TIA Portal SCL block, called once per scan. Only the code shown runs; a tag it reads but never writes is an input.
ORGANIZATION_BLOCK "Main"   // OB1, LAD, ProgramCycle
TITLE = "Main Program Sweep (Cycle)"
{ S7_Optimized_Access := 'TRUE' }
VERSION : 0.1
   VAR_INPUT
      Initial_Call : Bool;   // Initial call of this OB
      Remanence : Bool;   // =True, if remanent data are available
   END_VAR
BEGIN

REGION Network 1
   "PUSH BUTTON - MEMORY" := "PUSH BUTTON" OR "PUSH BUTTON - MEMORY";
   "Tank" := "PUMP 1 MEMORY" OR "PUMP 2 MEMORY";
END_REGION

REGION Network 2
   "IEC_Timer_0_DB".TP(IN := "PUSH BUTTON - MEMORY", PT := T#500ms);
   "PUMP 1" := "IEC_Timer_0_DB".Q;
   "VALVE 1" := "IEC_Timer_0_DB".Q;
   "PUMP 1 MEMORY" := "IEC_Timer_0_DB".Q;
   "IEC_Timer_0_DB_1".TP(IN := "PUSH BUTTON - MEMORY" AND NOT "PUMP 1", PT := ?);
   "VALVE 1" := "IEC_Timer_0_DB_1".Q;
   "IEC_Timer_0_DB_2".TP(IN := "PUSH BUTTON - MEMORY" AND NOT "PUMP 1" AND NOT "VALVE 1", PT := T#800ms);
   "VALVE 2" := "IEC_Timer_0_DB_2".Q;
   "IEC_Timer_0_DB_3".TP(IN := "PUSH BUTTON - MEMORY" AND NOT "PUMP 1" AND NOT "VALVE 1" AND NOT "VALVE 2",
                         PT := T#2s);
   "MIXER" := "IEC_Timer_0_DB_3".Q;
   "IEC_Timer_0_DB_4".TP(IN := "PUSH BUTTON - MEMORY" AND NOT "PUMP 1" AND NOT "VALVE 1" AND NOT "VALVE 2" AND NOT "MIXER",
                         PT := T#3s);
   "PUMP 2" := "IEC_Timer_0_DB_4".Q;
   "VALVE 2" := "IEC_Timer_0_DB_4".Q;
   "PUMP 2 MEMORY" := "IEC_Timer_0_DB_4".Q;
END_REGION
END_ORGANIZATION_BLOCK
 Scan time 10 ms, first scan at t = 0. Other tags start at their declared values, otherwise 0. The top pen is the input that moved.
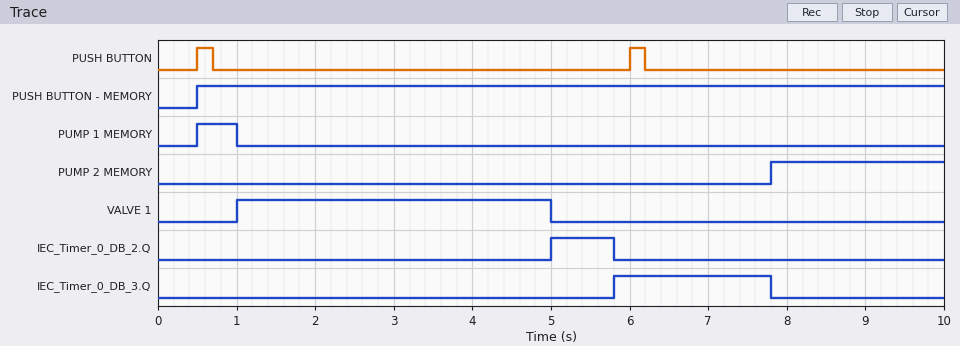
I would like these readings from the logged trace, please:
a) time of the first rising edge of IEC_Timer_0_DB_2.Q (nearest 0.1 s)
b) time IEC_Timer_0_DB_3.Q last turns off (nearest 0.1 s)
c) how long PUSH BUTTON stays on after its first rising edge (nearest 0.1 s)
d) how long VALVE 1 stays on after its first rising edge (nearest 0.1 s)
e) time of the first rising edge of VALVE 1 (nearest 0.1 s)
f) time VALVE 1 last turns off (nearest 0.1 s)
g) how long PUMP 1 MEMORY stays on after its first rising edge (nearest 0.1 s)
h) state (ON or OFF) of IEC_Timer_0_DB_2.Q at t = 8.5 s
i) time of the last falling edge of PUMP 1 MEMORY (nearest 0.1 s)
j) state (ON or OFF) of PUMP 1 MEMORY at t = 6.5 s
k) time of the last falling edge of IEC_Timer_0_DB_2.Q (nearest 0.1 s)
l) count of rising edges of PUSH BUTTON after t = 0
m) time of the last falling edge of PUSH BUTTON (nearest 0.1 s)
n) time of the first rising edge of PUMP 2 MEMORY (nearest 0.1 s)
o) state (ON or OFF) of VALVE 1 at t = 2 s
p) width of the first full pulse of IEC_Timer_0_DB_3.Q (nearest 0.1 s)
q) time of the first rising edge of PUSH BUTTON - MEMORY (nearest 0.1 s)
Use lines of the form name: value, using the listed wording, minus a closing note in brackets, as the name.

time of the first rising edge of IEC_Timer_0_DB_2.Q: 5.0 s
time IEC_Timer_0_DB_3.Q last turns off: 7.8 s
how long PUSH BUTTON stays on after its first rising edge: 0.2 s
how long VALVE 1 stays on after its first rising edge: 4.0 s
time of the first rising edge of VALVE 1: 1.0 s
time VALVE 1 last turns off: 5.0 s
how long PUMP 1 MEMORY stays on after its first rising edge: 0.5 s
state (ON or OFF) of IEC_Timer_0_DB_2.Q at t = 8.5 s: OFF
time of the last falling edge of PUMP 1 MEMORY: 1.0 s
state (ON or OFF) of PUMP 1 MEMORY at t = 6.5 s: OFF
time of the last falling edge of IEC_Timer_0_DB_2.Q: 5.8 s
count of rising edges of PUSH BUTTON after t = 0: 2
time of the last falling edge of PUSH BUTTON: 6.2 s
time of the first rising edge of PUMP 2 MEMORY: 7.8 s
state (ON or OFF) of VALVE 1 at t = 2 s: ON
width of the first full pulse of IEC_Timer_0_DB_3.Q: 2.0 s
time of the first rising edge of PUSH BUTTON - MEMORY: 0.5 s
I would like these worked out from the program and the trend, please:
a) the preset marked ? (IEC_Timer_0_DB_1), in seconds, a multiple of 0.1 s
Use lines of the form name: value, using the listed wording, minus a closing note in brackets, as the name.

the preset marked ? (IEC_Timer_0_DB_1), in seconds, a multiple of 0.1 s: 4.0 s
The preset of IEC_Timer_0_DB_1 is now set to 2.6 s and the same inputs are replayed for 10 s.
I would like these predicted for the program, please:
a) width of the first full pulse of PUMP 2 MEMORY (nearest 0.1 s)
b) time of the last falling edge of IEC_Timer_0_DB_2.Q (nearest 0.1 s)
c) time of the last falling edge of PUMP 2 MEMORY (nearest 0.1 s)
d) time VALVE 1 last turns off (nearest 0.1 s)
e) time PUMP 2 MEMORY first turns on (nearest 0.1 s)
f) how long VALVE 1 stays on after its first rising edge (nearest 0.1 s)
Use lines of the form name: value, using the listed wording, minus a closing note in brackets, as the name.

width of the first full pulse of PUMP 2 MEMORY: 3.0 s
time of the last falling edge of IEC_Timer_0_DB_2.Q: 4.4 s
time of the last falling edge of PUMP 2 MEMORY: 9.4 s
time VALVE 1 last turns off: 3.6 s
time PUMP 2 MEMORY first turns on: 6.4 s
how long VALVE 1 stays on after its first rising edge: 2.6 s
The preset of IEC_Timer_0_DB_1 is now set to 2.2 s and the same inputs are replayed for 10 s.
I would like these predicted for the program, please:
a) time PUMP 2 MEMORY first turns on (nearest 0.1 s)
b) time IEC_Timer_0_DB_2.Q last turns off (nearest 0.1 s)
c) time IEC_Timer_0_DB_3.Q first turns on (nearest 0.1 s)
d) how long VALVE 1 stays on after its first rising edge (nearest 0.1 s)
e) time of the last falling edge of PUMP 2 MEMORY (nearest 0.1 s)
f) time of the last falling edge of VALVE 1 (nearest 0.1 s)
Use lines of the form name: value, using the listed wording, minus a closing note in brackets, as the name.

time PUMP 2 MEMORY first turns on: 6.0 s
time IEC_Timer_0_DB_2.Q last turns off: 4.0 s
time IEC_Timer_0_DB_3.Q first turns on: 4.0 s
how long VALVE 1 stays on after its first rising edge: 2.2 s
time of the last falling edge of PUMP 2 MEMORY: 9.0 s
time of the last falling edge of VALVE 1: 3.2 s
